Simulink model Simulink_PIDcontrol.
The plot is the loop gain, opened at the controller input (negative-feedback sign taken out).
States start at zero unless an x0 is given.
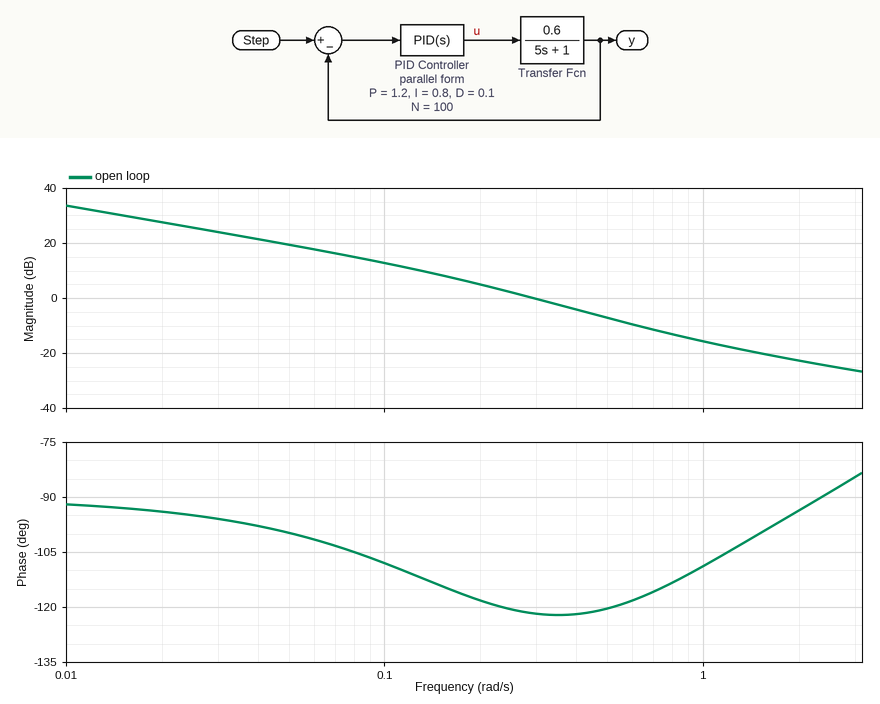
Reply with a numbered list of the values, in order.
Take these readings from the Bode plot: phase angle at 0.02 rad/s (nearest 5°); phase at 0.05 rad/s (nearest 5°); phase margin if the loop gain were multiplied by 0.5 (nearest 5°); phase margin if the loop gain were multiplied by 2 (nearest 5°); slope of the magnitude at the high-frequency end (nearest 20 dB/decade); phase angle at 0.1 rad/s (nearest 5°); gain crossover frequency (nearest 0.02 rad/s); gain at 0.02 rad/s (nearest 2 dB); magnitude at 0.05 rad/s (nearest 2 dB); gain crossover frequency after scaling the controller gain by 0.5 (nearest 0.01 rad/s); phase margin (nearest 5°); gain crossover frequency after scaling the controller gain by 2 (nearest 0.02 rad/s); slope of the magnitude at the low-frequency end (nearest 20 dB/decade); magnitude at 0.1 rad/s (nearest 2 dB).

1. -95°
2. -100°
3. 65°
4. 60°
5. -20 dB/decade
6. -110°
7. 0.30 rad/s
8. 28 dB
9. 20 dB
10. 0.18 rad/s
11. 60°
12. 0.46 rad/s
13. -20 dB/decade
14. 12 dB
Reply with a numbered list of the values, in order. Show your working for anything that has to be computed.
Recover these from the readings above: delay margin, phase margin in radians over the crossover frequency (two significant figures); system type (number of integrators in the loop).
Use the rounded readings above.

1. 60 × π / 180 / 0.3 = 3.5 s
2. 1
